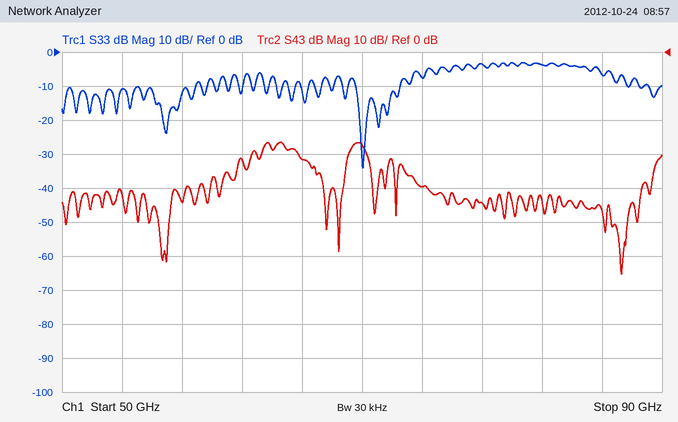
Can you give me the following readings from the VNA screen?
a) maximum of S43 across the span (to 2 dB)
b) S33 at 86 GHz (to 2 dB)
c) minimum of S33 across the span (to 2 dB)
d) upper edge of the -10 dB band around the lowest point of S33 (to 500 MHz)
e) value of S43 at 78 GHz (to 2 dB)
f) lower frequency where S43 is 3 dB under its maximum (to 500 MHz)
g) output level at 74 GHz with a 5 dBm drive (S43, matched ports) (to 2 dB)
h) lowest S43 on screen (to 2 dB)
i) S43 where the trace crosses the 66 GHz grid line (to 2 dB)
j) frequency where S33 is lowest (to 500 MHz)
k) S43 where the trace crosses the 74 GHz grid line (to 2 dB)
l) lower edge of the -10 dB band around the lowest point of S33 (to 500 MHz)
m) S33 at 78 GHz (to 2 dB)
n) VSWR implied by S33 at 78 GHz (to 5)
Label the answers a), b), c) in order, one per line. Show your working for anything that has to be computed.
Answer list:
a) -26 dB
b) -6 dB
c) -34 dB
d) 72.5 GHz
e) -44 dB
f) 63.5 GHz
g) 5 dBm + (-40 dB) = -34 dBm
h) -66 dB
i) -32 dB
j) 70.0 GHz
k) -40 dB
l) 69.5 GHz
m) -4 dB
n) |Γ| = 10^(-4/20) = 0.6310; VSWR = (1 + 0.6310)/(1 − 0.6310) ≈ 4.42, so 5 to the nearest 5
